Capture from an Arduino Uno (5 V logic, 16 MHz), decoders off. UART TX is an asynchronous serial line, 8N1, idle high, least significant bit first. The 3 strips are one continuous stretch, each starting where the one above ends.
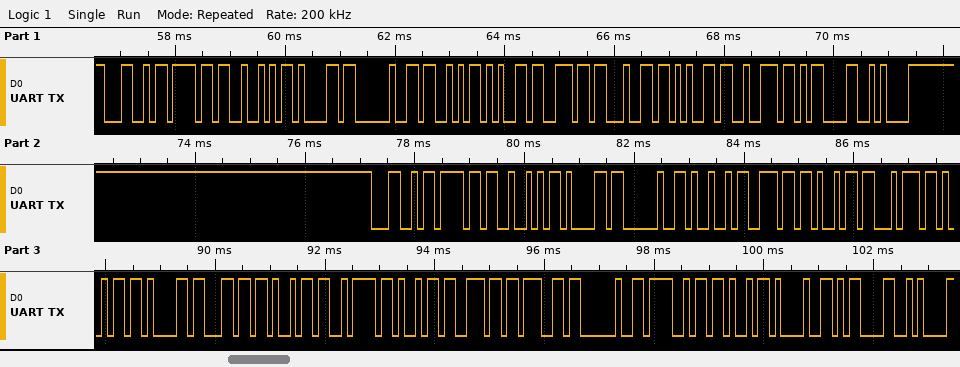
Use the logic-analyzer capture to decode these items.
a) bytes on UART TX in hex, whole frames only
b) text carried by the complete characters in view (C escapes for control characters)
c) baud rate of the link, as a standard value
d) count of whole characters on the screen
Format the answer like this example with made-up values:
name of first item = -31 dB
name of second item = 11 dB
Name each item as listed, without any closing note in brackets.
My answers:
bytes on UART TX in hex, whole frames only = 4C 6F 52 61 20 53 65 6E 64 65 72 0D 0A 4C 6F 52 61 20 49 6E 69 74 69 61 6C 69 7A 69 6E 67 20 4F 4B 21 0D 0A
text carried by the complete characters in view = "LoRa Sender\r\nLoRa Initializing OK!\r\n"
baud rate of the link, as a standard value = 9600 baud
count of whole characters on the screen = 36
